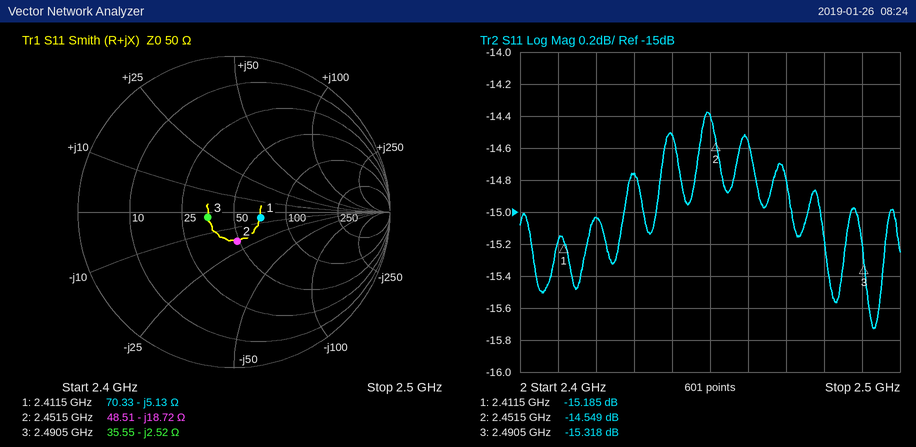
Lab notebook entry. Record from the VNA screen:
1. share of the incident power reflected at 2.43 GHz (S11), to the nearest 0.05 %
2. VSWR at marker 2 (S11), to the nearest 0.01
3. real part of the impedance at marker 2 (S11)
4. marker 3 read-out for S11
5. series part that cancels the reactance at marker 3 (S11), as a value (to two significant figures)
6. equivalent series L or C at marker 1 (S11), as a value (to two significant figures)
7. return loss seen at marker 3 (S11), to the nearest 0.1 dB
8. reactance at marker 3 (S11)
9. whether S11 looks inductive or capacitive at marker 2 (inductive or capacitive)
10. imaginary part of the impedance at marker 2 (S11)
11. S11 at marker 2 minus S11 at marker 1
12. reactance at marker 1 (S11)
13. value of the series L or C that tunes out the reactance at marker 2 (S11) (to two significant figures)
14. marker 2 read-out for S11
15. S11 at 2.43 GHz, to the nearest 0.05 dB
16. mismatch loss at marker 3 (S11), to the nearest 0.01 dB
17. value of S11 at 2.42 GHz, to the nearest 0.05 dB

3.35 %
1.46
48.51 Ω
-15.318 dB
160 pH
13 pF
15.3 dB
-2.52 Ω
capacitive
-18.72 Ω
0.636 dB
-5.13 Ω
1.2 nH
-14.549 dB
-14.75 dB
0.13 dB
-15.05 dB
